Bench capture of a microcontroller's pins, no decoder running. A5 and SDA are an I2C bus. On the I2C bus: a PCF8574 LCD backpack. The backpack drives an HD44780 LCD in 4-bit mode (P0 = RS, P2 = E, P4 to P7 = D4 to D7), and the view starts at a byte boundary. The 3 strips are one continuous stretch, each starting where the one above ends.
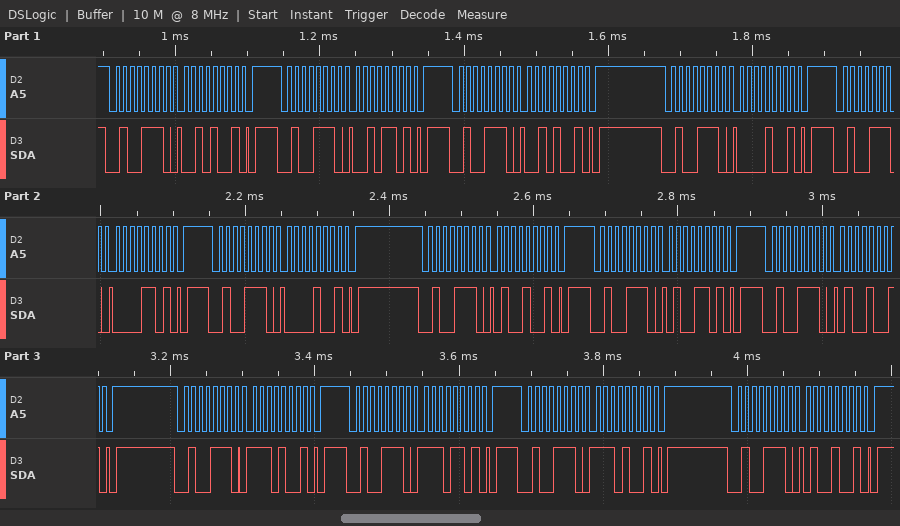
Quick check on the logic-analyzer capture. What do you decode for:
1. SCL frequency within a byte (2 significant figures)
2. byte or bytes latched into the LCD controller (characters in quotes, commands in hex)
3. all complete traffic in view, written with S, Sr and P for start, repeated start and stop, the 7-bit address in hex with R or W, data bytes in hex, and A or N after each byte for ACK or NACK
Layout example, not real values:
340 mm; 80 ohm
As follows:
100 kHz; ' ' 'N'; S 27W A 29 A P S 27W A 2D A P S 27W A 29 A P S 27W A 09 A P S 27W A 0D A P S 27W A 09 A P S 27W A 49 A P S 27W A 4D A P S 27W A 49 A P S 27W A E9 A P S 27W A ED A P S 27W A E9 A P S 27W A 49 A P
